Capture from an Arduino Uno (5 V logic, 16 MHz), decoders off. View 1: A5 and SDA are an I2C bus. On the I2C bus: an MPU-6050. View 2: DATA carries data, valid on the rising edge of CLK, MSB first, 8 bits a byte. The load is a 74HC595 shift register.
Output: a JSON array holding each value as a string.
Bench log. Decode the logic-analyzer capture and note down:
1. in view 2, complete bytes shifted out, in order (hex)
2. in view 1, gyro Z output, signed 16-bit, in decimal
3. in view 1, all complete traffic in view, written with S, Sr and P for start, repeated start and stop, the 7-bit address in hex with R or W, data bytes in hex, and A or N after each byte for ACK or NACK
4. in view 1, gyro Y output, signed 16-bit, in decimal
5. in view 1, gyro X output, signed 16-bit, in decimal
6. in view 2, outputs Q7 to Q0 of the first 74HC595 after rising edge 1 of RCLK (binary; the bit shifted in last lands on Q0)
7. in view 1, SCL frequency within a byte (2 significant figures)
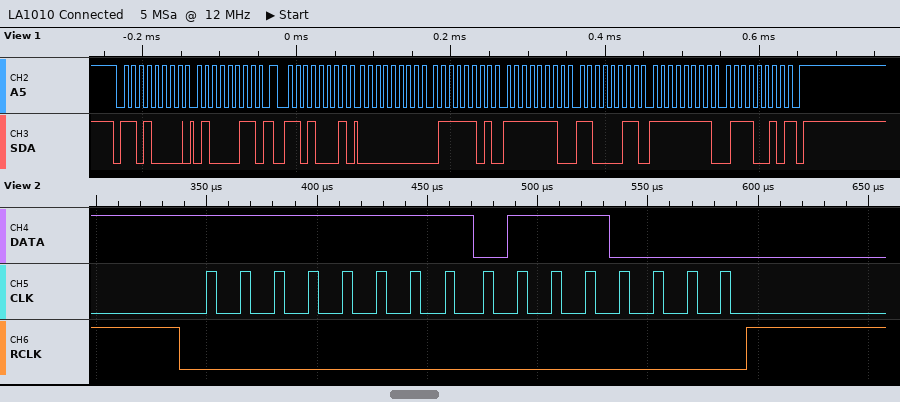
["0xFF 0x70", "-142", "S 68W A 43 A Sr 68R A 00 A 7D A FE A C3 A FF A 72 N P", "-317", "125", "01110000", "100 kHz"]
